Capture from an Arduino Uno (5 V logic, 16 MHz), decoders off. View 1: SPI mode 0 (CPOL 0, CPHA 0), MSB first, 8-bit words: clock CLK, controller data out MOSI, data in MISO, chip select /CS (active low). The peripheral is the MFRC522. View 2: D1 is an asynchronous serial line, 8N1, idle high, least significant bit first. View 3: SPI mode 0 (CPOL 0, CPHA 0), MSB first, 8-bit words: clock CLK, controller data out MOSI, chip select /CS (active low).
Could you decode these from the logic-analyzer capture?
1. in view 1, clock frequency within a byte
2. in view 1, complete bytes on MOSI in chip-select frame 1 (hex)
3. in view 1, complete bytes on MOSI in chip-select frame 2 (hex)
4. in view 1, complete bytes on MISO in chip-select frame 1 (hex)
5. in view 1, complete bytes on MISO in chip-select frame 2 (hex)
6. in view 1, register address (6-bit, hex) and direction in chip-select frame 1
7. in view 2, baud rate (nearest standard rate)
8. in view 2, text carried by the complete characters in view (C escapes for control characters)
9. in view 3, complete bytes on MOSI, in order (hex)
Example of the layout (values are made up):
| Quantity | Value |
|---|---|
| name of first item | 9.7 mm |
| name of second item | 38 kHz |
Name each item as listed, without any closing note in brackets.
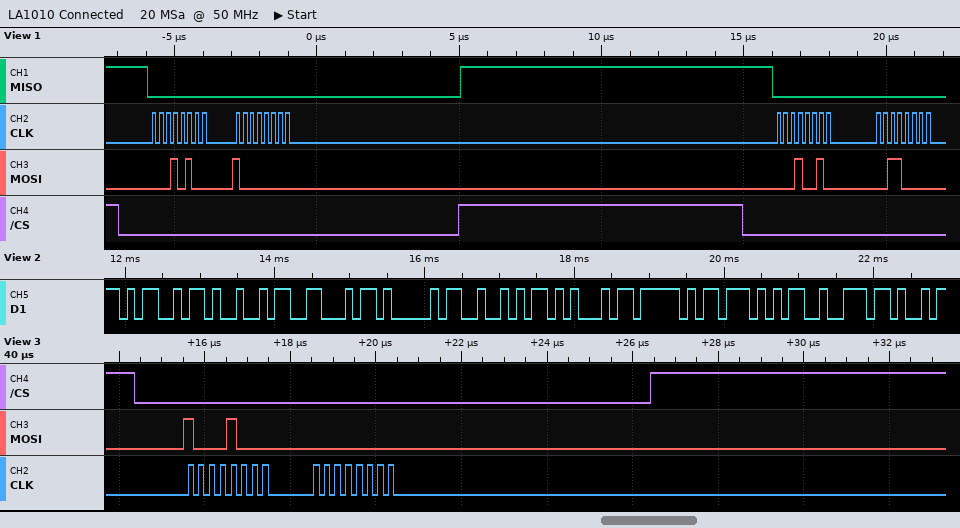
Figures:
| Quantity | Value |
|---|---|
| in view 1, clock frequency within a byte | 4 MHz |
| in view 1, complete bytes on MOSI in chip-select frame 1 | 0x14 0x80 |
| in view 1, complete bytes on MOSI in chip-select frame 2 | 0x12 0x30 |
| in view 1, complete bytes on MISO in chip-select frame 1 | 0x00 0x00 |
| in view 1, complete bytes on MISO in chip-select frame 2 | 0x00 0x00 |
| in view 1, register address (6-bit, hex) and direction in chip-select frame 1 | 0x0A write |
| in view 2, baud rate | 9600 baud |
| in view 2, text carried by the complete characters in view | "MIFARE_Wr" |
| in view 3, complete bytes on MOSI, in order | 88 00 |
